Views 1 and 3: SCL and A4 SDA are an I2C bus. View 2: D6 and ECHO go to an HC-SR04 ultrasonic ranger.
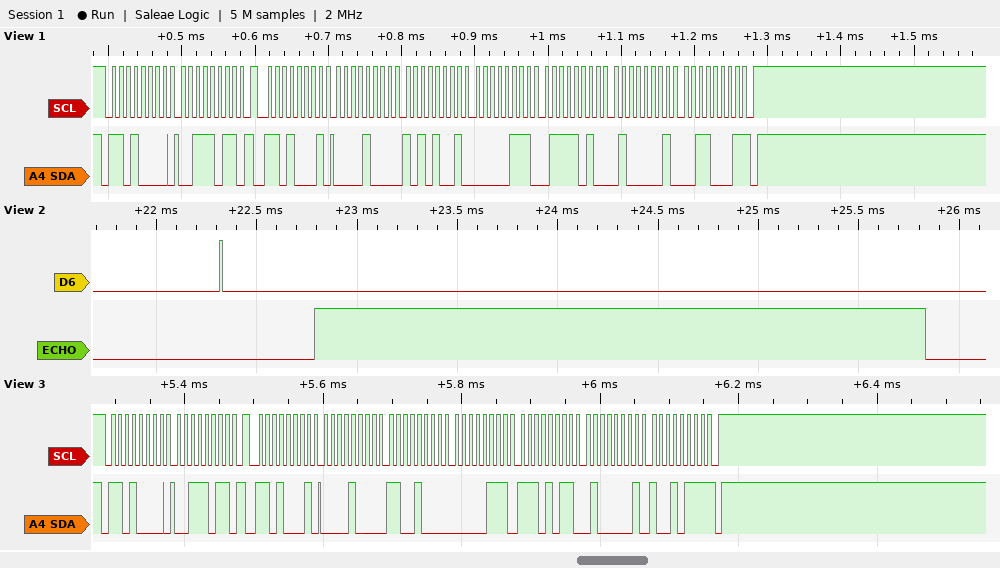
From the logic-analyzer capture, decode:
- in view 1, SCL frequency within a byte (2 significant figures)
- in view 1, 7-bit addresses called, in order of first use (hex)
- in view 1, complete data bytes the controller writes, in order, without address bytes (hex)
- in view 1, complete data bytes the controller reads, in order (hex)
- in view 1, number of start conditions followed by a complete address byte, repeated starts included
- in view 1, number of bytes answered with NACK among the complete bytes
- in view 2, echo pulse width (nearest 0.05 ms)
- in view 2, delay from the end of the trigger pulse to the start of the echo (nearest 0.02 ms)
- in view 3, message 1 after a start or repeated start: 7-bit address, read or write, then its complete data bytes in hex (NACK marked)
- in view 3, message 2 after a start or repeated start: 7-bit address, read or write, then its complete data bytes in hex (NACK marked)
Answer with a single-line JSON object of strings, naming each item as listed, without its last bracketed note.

{"in view 1, SCL frequency within a byte": "100 kHz", "in view 1, 7-bit addresses called, in order of first use": "0x68", "in view 1, complete data bytes the controller writes, in order, without address bytes": "3B", "in view 1, complete data bytes the controller reads, in order": "08 A9 07 7A 41 31", "in view 1, number of start conditions followed by a complete address byte, repeated starts included": "2", "in view 1, number of bytes answered with NACK among the complete bytes": "1", "in view 2, echo pulse width": "3.05 ms", "in view 2, delay from the end of the trigger pulse to the start of the echo": "0.46 ms", "in view 3, message 1 after a start or repeated start: 7-bit address, read or write, then its complete data bytes in hex": "0x68 write: 3B", "in view 3, message 2 after a start or repeated start: 7-bit address, read or write, then its complete data bytes in hex": "0x68 read: 08 C8 07 EB 41 97 NACK"}
